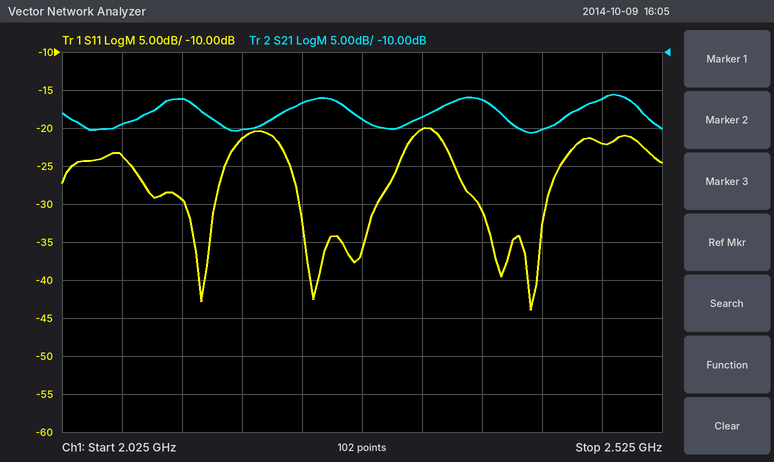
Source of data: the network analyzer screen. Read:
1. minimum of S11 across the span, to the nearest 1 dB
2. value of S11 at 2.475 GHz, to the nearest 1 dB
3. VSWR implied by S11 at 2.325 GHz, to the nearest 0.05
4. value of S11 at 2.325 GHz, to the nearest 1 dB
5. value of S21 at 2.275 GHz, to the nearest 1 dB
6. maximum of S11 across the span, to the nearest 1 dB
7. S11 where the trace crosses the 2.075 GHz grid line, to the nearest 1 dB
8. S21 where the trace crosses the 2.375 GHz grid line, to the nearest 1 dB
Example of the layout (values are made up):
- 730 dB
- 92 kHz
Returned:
- -44 dB
- -22 dB
- 1.20
- -20 dB
- -19 dB
- -20 dB
- -24 dB
- -16 dB
